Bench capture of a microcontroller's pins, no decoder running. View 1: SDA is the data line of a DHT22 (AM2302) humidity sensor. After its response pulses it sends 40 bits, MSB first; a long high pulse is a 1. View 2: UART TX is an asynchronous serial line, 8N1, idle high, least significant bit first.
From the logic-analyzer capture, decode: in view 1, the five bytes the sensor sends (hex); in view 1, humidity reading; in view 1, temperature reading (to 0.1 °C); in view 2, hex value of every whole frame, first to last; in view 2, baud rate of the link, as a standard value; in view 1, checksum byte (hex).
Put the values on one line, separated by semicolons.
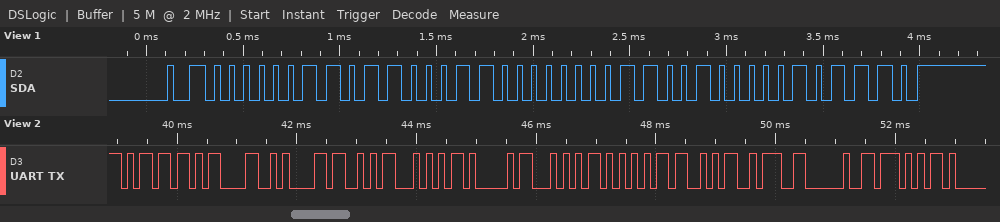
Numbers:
03 63 00 C8 2E; 86.7 %; 20.0 °C; 6D 0D 0A 53 54 41 54 55 53 3A 20 57; 9600 baud; 0x2E
